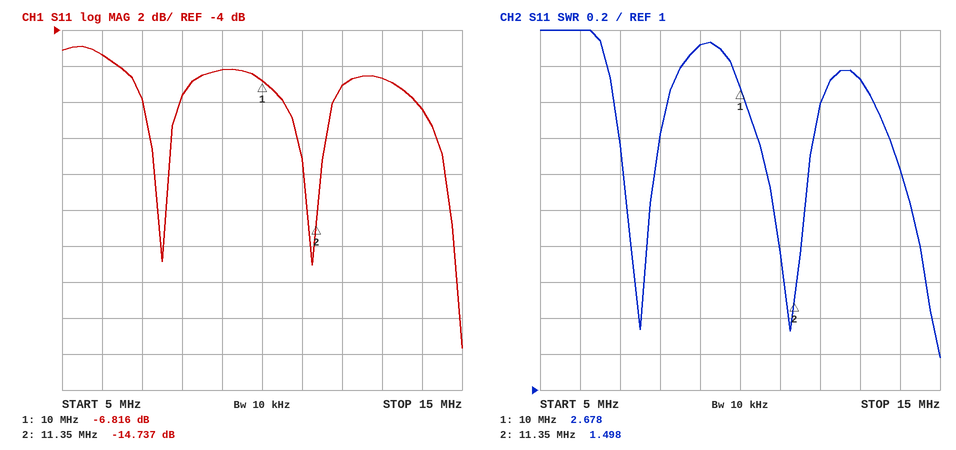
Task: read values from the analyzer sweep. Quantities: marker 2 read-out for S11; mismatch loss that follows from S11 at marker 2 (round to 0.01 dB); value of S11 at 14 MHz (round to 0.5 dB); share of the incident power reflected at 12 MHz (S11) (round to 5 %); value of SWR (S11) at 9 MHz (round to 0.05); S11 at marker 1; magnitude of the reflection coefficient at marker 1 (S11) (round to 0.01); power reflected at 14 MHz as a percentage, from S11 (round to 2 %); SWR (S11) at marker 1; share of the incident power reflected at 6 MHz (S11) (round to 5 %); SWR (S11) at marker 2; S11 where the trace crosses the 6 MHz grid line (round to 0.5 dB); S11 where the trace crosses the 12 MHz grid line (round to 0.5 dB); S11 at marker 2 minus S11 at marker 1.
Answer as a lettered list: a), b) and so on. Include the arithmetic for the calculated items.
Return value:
a) -14.737 dB
b) −10 log10(1 − 10^(-14.737/10)) ≈ 0.15 dB
c) -8.5 dB
d) 10^(-7/10) ≈ 20 %
e) 2.90
f) -6.816 dB
g) 10^(-6.816/20) ≈ 0.46
h) 10^(-8.5/10) ≈ 14 %
i) 2.678
j) 10^(-5.5/10) ≈ 28.2 %, so 30 % to the nearest 5 %
k) 1.498
l) -5.5 dB
m) -7.0 dB
n) -14.737 − (-6.816) = -7.921 dB
